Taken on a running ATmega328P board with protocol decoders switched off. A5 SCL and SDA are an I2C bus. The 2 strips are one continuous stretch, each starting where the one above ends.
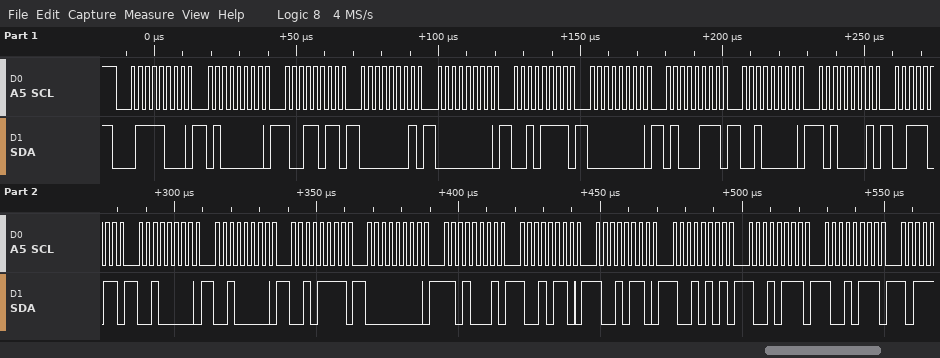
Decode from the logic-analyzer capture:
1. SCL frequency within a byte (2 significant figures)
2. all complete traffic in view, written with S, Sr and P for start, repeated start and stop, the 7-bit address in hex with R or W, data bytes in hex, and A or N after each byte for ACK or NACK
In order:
400 kHz
S 3CW A 40 A 9B A 01 A 00 A 2F A 00 A 47 A 20 A A1 A 3B A 20 A 20 A 2F A 00 A D1 A 96 A 96 A 95 A 97 A 97 A
